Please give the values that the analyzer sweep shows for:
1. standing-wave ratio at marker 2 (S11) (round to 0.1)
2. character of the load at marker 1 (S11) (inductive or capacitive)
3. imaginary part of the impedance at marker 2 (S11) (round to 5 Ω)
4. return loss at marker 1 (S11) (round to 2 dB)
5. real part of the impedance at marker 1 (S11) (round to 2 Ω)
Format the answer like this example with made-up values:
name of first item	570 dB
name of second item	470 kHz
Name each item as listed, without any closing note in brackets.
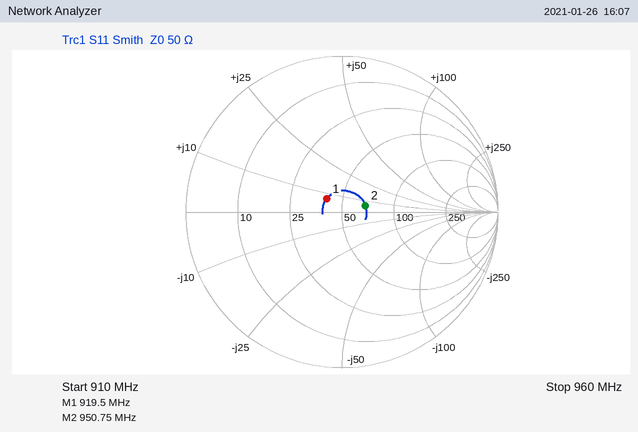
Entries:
standing-wave ratio at marker 2 (S11)	1.4
character of the load at marker 1 (S11)	inductive
imaginary part of the impedance at marker 2 (S11)	+5 Ω
return loss at marker 1 (S11)	18 dB
real part of the impedance at marker 1 (S11)	40 Ω
